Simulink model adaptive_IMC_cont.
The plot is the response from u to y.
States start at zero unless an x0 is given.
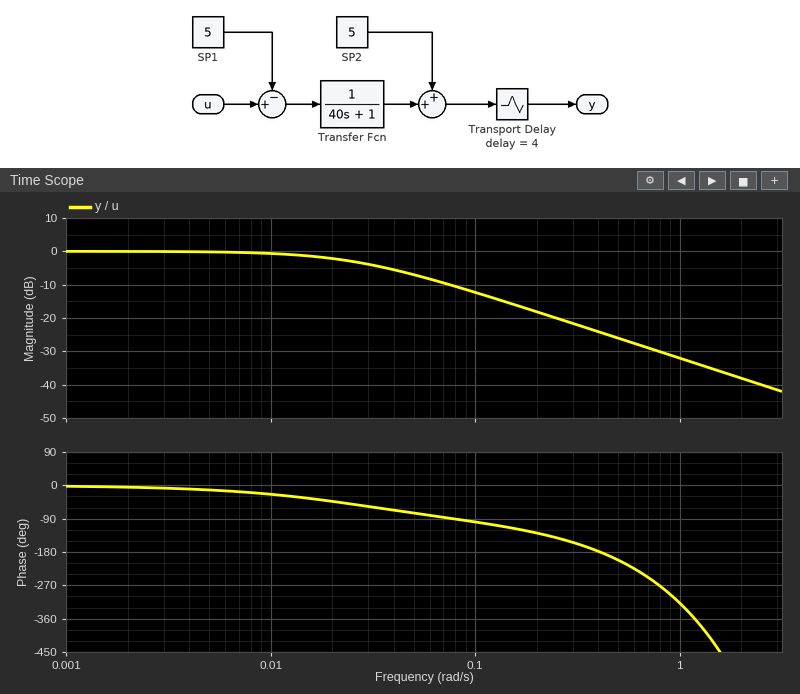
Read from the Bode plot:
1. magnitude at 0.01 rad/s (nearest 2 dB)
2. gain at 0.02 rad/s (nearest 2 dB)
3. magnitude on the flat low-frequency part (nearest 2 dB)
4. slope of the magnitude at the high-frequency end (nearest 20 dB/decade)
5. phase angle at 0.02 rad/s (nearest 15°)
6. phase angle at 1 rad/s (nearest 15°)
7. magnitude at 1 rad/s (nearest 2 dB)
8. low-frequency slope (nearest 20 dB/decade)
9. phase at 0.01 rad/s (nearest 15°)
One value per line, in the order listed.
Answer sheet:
0 dB
-2 dB
0 dB
-20 dB/decade
-45°
-315°
-32 dB
0 dB/decade
-30°
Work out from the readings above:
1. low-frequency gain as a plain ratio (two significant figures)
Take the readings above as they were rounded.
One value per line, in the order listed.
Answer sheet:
1.0
